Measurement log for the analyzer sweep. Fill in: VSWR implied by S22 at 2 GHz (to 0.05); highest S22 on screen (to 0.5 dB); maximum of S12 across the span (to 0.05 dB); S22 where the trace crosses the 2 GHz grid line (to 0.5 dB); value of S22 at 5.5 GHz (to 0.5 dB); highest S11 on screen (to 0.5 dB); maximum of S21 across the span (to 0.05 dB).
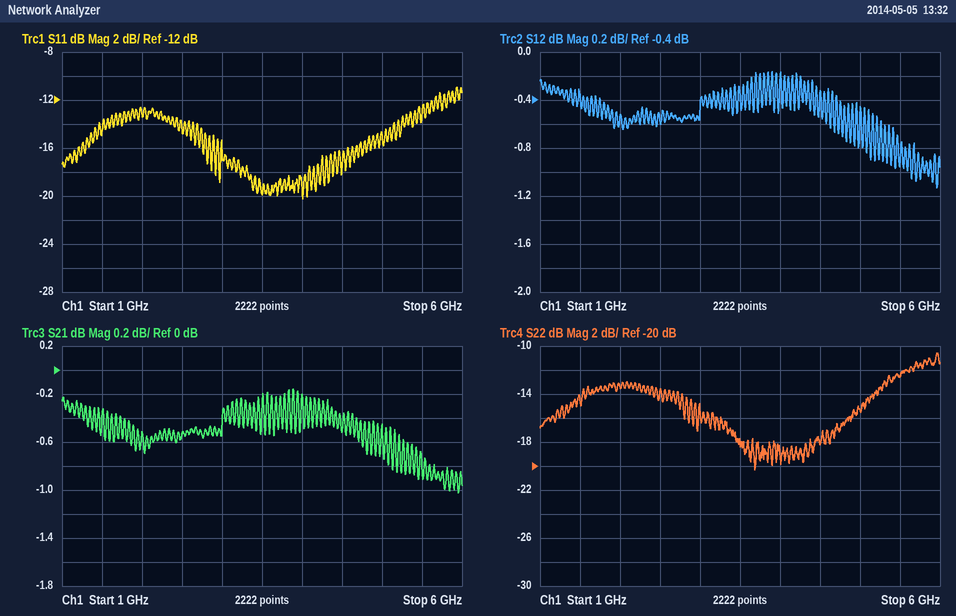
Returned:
1.55
-10.5 dB
-0.15 dB
-13.5 dB
-12.5 dB
-11.0 dB
-0.15 dB
